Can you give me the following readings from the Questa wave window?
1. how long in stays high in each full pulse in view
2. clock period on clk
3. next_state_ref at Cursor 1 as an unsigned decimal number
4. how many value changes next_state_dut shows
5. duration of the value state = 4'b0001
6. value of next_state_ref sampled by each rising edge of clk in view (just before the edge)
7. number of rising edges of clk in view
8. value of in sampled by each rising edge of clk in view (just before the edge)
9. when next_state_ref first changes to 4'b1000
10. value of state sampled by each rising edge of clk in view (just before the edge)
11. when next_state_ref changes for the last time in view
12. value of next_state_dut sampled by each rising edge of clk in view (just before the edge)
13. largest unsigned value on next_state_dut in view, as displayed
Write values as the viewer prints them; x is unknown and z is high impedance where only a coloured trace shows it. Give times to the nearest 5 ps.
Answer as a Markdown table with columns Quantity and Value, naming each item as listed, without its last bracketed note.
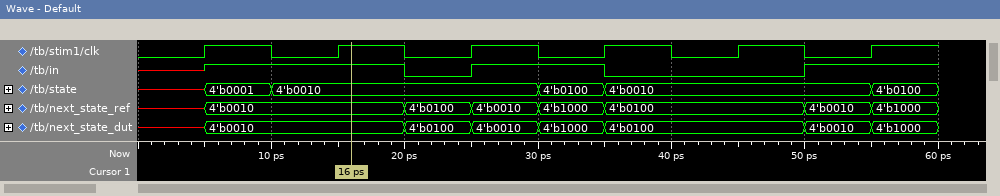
| Quantity | Value |
|---|---|
| how long in stays high in each full pulse in view | 10 ps |
| clock period on clk | 10 ps |
| next_state_ref at Cursor 1 as an unsigned decimal number | 2 |
| how many value changes next_state_dut shows | 7 |
| duration of the value state = 4'b0001 | 5 ps |
| value of next_state_ref sampled by each rising edge of clk in view | x, 4'b0010, 4'b0100, 4'b1000, 4'b0100, 4'b0010 |
| number of rising edges of clk in view | 6 |
| value of in sampled by each rising edge of clk in view | x 1 0 1 0 1 |
| when next_state_ref first changes to 4'b1000 | 30 ps |
| value of state sampled by each rising edge of clk in view | x, 4'b0010, 4'b0010, 4'b0100, 4'b0010, 4'b0010 |
| when next_state_ref changes for the last time in view | 55 ps |
| value of next_state_dut sampled by each rising edge of clk in view | x, 4'b0010, 4'b0100, 4'b1000, 4'b0100, 4'b0010 |
| largest unsigned value on next_state_dut in view, as displayed | 4'b1000 |
